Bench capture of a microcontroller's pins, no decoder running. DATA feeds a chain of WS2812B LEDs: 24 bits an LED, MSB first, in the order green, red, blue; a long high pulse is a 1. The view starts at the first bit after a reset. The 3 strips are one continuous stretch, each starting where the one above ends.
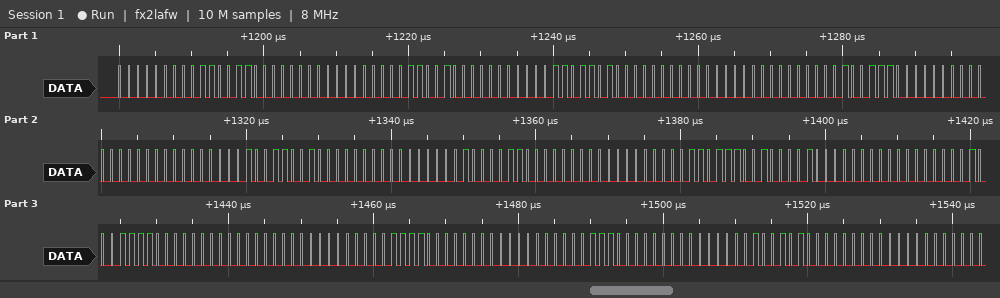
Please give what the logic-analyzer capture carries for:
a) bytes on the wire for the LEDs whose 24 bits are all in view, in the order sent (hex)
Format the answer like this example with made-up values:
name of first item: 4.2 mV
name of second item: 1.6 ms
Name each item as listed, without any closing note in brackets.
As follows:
bytes on the wire for the LEDs whose 24 bits are all in view, in the order sent: 00 66 00 00 C8 00 DA 00 00 00 9C 00 00 00 99 00 00 86 00 00 6E 42 00 00 8F 00 00 00 3C 00 00 E0 00 25 00 00
